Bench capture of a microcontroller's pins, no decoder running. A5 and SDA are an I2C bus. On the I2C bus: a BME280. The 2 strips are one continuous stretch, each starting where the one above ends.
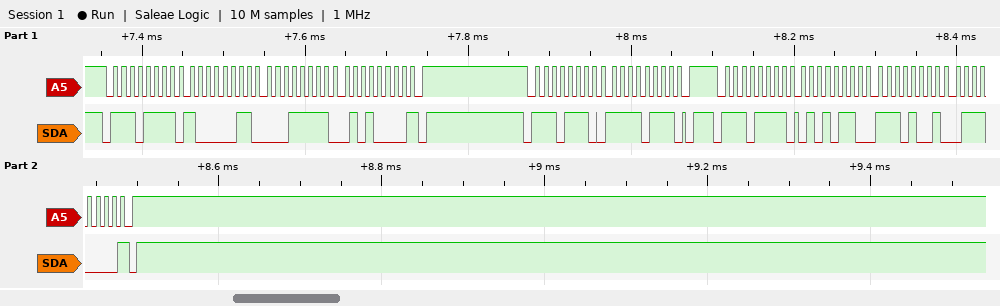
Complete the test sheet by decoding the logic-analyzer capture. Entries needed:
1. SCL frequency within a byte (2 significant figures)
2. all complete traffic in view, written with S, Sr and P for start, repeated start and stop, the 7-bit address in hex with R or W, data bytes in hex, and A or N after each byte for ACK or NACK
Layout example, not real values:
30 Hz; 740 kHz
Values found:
100 kHz; S 77R A 83 A 1F A 50 N P S 77W A F7 A P S 77R A 56 A E9 A 70 N P
